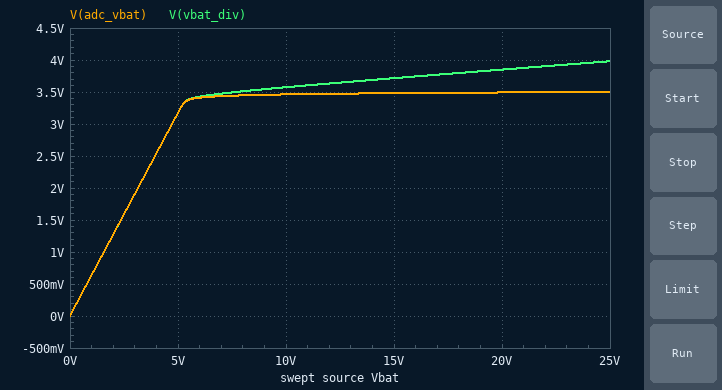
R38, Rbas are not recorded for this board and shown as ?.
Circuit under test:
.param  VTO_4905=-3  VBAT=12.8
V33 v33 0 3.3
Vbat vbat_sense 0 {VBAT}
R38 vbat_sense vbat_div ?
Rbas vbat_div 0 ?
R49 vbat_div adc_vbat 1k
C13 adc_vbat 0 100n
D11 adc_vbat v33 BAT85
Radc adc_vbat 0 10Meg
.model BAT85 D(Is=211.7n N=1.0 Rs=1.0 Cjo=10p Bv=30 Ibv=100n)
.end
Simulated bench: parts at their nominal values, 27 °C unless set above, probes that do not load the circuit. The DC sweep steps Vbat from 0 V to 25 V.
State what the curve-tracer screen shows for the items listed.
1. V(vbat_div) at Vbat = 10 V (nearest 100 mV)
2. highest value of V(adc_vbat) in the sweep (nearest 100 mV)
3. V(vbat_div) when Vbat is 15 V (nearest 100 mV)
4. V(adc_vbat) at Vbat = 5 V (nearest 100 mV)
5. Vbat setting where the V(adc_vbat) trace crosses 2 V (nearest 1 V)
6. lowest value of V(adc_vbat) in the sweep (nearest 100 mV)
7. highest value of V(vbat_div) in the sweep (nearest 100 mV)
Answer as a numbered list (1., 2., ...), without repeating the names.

1. 3.6 V
2. 3.5 V
3. 3.7 V
4. 3.2 V
5. 3 V
6. 0 V
7. 4.0 V
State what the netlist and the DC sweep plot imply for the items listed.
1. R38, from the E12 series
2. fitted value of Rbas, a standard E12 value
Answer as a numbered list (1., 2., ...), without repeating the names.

1. 39 kΩ
2. 68 kΩ
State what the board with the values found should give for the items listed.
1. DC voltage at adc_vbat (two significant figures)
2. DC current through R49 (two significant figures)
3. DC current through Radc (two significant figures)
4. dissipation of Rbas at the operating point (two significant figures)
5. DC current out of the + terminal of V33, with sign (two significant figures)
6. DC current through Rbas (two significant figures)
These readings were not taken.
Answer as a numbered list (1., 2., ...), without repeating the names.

1. 3.5 V
2. 180 µA
3. 350 nA
4. 200 µW
5. -180 µA
6. 54 µA
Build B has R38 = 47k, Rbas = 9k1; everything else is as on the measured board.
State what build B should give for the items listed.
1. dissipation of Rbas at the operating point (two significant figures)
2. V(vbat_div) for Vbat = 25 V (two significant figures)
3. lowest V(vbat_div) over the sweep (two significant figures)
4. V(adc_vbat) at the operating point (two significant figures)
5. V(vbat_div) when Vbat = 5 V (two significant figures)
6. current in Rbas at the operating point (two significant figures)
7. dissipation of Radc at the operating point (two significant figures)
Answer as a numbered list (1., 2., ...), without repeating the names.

1. 470 µW
2. 3.5 V
3. 1.6 mV
4. 2.1 V
5. 810 mV
6. 230 µA
7. 430 nW
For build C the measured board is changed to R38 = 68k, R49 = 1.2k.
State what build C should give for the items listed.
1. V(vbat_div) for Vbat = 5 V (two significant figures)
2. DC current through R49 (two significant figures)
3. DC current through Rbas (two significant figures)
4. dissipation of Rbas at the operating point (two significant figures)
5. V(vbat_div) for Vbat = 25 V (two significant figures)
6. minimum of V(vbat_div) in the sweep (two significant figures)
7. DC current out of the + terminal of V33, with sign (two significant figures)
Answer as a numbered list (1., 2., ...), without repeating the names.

1. 2.5 V
2. 84 µA
3. 52 µA
4. 190 µW
5. 3.8 V
6. 7.2 mV
7. -83 µA
